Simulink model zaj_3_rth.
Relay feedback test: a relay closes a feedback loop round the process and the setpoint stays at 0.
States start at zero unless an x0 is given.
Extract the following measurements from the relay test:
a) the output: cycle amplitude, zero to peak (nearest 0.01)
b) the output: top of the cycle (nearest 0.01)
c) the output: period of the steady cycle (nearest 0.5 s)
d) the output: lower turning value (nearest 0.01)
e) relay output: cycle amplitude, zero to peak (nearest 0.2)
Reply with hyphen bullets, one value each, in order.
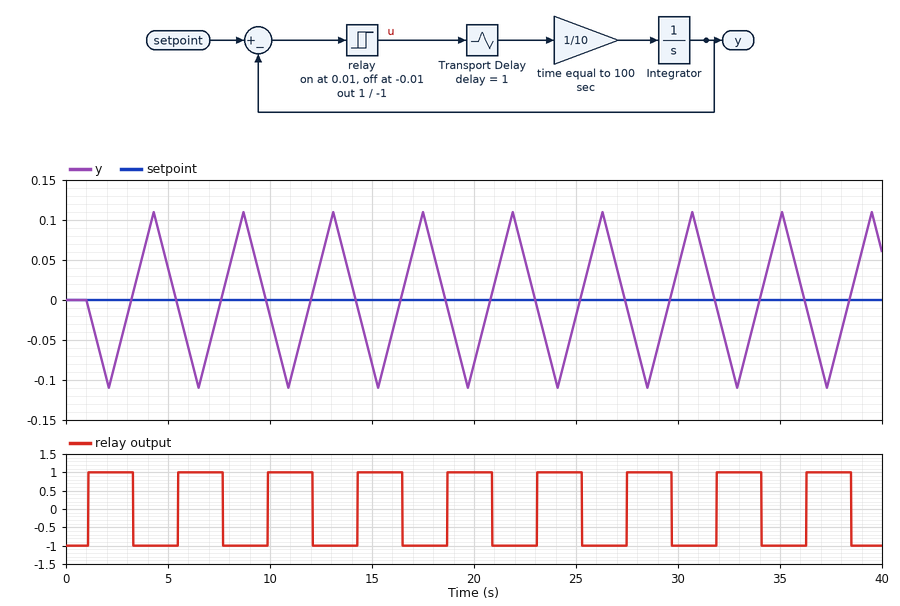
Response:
- 0.11
- 0.11
- 4.5 s
- -0.11
- 1.0
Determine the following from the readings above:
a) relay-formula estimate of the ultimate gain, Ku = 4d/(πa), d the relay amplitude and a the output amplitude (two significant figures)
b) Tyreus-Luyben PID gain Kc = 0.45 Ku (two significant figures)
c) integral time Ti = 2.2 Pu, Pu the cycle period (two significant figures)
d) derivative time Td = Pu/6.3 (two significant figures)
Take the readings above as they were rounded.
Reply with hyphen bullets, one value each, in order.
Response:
- 12
- 5.4
- 9.9 s
- 0.71 s
